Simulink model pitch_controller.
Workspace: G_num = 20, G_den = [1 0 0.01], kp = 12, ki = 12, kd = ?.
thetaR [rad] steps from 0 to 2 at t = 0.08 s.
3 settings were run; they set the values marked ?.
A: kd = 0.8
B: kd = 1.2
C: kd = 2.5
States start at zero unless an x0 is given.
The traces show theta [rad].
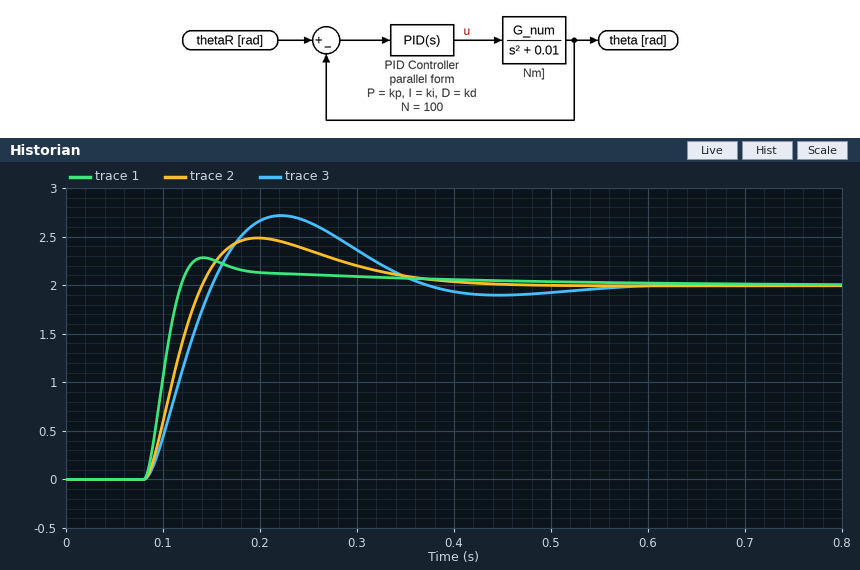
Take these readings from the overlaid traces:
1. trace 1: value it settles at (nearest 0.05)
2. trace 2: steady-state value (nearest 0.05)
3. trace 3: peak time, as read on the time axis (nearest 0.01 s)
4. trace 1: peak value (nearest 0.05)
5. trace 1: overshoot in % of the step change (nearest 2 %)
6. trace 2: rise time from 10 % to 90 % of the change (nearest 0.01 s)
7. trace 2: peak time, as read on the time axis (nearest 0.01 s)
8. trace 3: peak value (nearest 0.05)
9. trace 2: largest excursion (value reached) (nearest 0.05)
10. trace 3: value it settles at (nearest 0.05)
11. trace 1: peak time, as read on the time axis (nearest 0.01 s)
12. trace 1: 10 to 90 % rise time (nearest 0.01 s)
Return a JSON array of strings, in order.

["2.00", "2.00", "0.22 s", "2.30", "14 %", "0.04 s", "0.20 s", "2.70", "2.50", "2.00", "0.14 s", "0.03 s"]
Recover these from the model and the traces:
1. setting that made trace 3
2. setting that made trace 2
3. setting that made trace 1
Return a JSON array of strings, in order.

["A", "B", "C"]
